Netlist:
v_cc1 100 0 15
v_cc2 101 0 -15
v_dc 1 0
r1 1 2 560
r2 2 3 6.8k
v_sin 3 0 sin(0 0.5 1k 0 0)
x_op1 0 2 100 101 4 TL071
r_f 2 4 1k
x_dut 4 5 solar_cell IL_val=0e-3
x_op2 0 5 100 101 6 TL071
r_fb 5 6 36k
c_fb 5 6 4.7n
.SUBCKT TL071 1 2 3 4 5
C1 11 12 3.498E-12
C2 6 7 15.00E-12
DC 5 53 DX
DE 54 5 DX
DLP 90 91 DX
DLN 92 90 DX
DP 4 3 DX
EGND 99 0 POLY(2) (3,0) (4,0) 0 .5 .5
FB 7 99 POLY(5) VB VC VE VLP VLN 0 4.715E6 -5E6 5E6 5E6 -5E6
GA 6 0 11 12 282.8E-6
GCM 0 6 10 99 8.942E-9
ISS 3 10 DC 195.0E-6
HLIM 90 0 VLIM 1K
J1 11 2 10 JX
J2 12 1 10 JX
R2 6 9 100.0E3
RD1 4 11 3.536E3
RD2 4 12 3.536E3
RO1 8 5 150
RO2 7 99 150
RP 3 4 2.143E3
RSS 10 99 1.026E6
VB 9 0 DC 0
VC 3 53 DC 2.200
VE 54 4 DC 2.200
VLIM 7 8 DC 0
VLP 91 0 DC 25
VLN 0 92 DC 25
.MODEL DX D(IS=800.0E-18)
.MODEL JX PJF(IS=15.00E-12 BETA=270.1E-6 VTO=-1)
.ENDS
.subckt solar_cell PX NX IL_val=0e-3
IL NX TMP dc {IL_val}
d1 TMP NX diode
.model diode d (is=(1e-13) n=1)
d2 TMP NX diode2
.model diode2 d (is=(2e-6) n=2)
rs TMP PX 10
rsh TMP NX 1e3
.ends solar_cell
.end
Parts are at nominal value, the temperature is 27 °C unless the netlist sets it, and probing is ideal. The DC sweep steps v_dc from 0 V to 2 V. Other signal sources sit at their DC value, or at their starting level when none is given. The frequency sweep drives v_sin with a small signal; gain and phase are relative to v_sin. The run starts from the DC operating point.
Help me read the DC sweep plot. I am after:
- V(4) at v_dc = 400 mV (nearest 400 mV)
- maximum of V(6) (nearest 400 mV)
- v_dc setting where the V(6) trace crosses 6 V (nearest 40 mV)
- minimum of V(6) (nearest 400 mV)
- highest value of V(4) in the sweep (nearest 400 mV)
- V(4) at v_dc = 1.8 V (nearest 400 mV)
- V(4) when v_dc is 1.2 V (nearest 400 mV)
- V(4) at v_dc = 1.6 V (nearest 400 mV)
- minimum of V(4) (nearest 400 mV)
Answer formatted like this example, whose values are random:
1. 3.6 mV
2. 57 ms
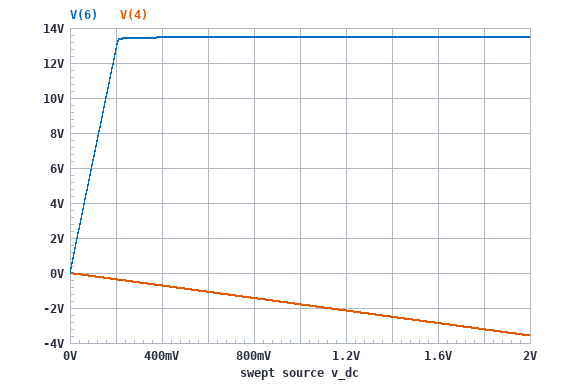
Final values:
1. -800 mV
2. 13.6 V
3. 80 mV
4. 0 V
5. 0 V
6. -3.2 V
7. -2.0 V
8. -2.8 V
9. -3.6 V
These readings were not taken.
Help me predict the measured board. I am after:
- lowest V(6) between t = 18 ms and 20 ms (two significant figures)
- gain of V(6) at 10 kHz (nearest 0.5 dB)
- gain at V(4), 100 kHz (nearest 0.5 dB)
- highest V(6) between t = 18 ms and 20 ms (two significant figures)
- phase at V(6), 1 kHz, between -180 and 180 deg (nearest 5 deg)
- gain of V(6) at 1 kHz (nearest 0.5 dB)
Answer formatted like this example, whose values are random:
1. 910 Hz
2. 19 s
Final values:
1. -1.9 V
2. -6.0 dB
3. -16.5 dB
4. 1.8 V
5. -45 deg
6. 11.5 dB
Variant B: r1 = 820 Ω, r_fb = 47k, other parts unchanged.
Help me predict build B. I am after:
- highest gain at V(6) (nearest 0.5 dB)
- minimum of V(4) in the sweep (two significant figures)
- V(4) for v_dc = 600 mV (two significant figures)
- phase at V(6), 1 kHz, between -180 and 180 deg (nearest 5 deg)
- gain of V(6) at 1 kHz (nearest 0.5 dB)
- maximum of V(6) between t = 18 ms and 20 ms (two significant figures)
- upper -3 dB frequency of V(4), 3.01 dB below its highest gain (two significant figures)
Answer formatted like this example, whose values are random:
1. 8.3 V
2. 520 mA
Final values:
1. 17.0 dB
2. -2.4 V
3. -730 mV
4. -55 deg
5. 12.5 dB
6. 2.0 V
7. 1.5 MHz
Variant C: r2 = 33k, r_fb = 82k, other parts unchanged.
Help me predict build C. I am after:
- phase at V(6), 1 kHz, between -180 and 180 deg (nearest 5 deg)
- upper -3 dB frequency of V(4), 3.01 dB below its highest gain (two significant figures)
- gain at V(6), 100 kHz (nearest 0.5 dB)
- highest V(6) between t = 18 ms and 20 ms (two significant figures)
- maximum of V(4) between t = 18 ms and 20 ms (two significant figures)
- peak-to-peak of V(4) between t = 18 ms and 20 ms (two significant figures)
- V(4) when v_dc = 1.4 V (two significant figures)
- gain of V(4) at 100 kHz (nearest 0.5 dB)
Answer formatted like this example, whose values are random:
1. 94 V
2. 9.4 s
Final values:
1. -70 deg
2. 1.2 MHz
3. -39.5 dB
4. 480 mV
5. 15 mV
6. 30 mV
7. -2.5 V
8. -30.5 dB
